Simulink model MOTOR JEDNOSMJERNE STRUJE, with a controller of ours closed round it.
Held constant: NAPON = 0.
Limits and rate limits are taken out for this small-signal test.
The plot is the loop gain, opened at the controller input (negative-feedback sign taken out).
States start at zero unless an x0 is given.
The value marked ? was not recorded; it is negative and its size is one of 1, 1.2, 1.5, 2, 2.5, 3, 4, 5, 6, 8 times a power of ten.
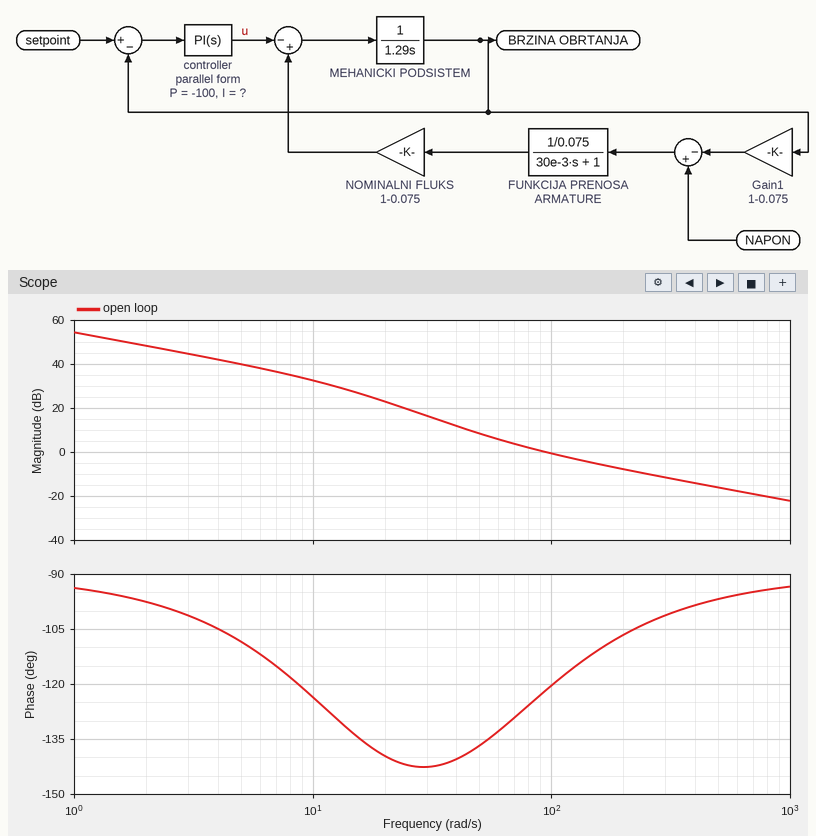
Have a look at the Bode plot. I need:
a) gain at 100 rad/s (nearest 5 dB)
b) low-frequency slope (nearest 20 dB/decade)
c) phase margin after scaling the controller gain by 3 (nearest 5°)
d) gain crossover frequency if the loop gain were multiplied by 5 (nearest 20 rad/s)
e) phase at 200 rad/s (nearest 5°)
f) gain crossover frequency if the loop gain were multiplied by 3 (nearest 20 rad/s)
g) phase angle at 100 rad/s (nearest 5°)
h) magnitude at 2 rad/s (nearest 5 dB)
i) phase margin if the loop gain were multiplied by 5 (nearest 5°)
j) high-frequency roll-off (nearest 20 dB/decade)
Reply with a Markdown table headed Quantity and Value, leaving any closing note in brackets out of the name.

| Quantity | Value |
|---|---|
| gain at 100 rad/s | 0 dB |
| low-frequency slope | -20 dB/decade |
| phase margin after scaling the controller gain by 3 | 75° |
| gain crossover frequency if the loop gain were multiplied by 5 | 400 rad/s |
| phase at 200 rad/s | -105° |
| gain crossover frequency if the loop gain were multiplied by 3 | 240 rad/s |
| phase angle at 100 rad/s | -120° |
| magnitude at 2 rad/s | 50 dB |
| phase margin if the loop gain were multiplied by 5 | 80° |
| high-frequency roll-off | -20 dB/decade |
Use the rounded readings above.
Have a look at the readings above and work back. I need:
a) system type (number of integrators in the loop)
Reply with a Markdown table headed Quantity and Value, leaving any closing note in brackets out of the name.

| Quantity | Value |
|---|---|
| system type | 1 |
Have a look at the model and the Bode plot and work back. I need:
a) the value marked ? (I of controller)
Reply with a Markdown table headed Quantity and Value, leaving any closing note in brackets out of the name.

| Quantity | Value |
|---|---|
| the value marked ? | -6000 |
